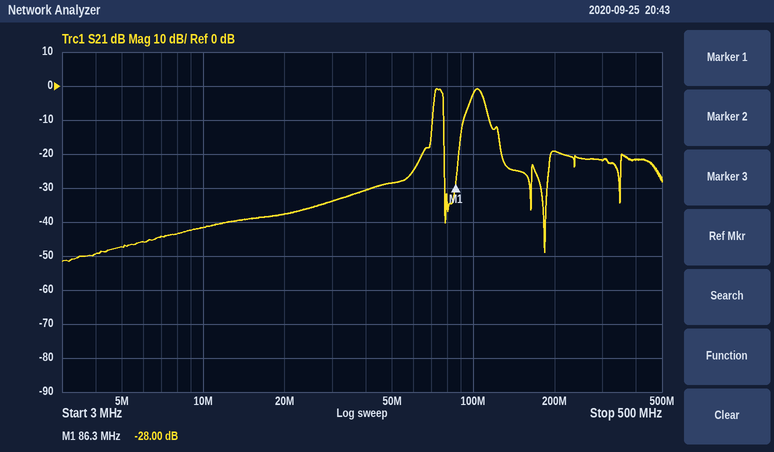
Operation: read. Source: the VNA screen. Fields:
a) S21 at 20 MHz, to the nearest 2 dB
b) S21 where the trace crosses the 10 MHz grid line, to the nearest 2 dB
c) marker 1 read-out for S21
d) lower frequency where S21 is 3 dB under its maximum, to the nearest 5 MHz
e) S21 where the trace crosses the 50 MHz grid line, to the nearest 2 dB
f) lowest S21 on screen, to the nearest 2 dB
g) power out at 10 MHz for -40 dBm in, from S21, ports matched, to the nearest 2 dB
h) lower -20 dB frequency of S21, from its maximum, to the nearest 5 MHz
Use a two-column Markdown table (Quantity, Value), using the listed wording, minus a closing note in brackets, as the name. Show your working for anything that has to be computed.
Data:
| Quantity | Value |
|---|---|
| S21 at 20 MHz, to the nearest 2 dB | -38 dB |
| S21 where the trace crosses the 10 MHz grid line, to the nearest 2 dB | -42 dB |
| marker 1 read-out for S21 | -28.00 dB |
| lower frequency where S21 is 3 dB under its maximum, to the nearest 5 MHz | 70 MHz |
| S21 where the trace crosses the 50 MHz grid line, to the nearest 2 dB | -28 dB |
| lowest S21 on screen, to the nearest 2 dB | -52 dB |
| power out at 10 MHz for -40 dBm in, from S21, ports matched, to the nearest 2 dB | -40 dBm + (-42 dB) = -82 dBm |
| lower -20 dB frequency of S21, from its maximum, to the nearest 5 MHz | 65 MHz |
